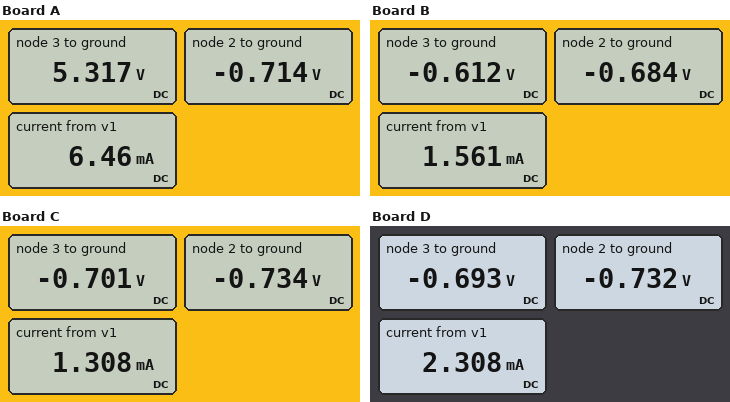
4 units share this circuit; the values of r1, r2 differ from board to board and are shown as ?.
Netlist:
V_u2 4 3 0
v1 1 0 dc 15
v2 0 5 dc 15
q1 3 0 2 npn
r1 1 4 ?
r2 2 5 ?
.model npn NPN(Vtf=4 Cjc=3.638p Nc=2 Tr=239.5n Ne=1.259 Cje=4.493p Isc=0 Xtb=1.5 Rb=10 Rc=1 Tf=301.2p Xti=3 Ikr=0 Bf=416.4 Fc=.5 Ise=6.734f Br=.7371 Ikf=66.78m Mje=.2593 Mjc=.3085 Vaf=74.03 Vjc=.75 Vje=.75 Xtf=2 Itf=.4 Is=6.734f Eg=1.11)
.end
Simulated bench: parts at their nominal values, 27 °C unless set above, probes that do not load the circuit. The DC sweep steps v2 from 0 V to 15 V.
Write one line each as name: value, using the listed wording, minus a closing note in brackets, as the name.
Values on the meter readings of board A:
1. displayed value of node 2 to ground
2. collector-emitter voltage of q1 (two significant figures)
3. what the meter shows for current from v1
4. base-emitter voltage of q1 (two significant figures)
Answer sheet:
displayed value of node 2 to ground: -0.714 V
collector-emitter voltage of q1: 6.0 V
what the meter shows for current from v1: 6.46 mA
base-emitter voltage of q1: 710 mV
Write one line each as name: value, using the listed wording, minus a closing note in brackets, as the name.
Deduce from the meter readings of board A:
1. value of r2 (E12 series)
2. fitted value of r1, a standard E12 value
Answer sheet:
value of r2: 2.2 kΩ
fitted value of r1, a standard E12 value: 1.5 kΩ
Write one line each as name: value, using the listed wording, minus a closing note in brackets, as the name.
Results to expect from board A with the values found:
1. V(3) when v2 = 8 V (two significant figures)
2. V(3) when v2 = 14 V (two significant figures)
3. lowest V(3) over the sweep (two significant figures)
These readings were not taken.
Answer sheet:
V(3) when v2 = 8 V: 10 V
V(3) when v2 = 14 V: 6.0 V
lowest V(3) over the sweep: 5.3 V
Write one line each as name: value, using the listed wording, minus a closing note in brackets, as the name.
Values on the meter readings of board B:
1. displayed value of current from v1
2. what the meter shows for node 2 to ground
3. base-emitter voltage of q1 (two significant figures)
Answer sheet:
displayed value of current from v1: 1.561 mA
what the meter shows for node 2 to ground: -0.684 V
base-emitter voltage of q1: 680 mV
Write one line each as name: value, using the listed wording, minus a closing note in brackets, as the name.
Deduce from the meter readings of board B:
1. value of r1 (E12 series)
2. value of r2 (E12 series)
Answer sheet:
value of r1: 10 kΩ
value of r2: 8.2 kΩ
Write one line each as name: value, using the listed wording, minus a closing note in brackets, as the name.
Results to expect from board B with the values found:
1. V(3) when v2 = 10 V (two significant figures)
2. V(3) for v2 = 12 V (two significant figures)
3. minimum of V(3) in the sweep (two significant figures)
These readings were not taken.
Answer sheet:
V(3) when v2 = 10 V: 3.7 V
V(3) for v2 = 12 V: 1.3 V
minimum of V(3) in the sweep: -610 mV
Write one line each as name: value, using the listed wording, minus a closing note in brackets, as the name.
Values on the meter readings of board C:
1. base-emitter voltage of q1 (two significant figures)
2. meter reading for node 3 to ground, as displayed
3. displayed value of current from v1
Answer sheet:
base-emitter voltage of q1: 730 mV
meter reading for node 3 to ground, as displayed: -0.701 V
displayed value of current from v1: 1.308 mA
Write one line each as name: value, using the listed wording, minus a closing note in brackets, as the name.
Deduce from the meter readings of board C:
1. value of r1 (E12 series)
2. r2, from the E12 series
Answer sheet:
value of r1: 12 kΩ
r2, from the E12 series: 3.9 kΩ
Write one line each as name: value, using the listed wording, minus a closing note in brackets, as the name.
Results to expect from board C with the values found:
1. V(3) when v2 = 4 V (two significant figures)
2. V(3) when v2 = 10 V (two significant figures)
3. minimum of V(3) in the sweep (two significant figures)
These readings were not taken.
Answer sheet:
V(3) when v2 = 4 V: 4.8 V
V(3) when v2 = 10 V: -670 mV
minimum of V(3) in the sweep: -700 mV
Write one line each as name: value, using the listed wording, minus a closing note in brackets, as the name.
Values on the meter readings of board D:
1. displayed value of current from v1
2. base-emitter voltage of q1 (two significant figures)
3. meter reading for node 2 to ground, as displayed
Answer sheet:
displayed value of current from v1: 2.308 mA
base-emitter voltage of q1: 730 mV
meter reading for node 2 to ground, as displayed: -0.732 V
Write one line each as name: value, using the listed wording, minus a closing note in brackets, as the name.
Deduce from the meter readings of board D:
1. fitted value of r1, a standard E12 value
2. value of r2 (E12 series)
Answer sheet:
fitted value of r1, a standard E12 value: 6.8 kΩ
value of r2: 3.3 kΩ
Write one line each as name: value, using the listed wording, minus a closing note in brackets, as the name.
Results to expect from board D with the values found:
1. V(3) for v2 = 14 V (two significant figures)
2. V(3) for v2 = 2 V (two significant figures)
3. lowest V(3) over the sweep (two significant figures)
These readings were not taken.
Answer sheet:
V(3) for v2 = 14 V: -690 mV
V(3) for v2 = 2 V: 12 V
lowest V(3) over the sweep: -690 mV
